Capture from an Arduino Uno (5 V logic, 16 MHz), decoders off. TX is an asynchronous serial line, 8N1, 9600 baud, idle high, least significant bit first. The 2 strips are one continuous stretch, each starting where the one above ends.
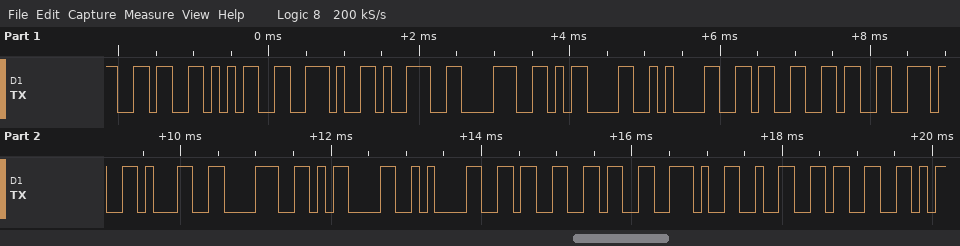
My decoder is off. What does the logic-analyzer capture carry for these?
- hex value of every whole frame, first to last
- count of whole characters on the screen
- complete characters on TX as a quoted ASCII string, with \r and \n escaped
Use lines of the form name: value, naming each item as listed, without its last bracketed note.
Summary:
hex value of every whole frame, first to last: 36 35 2E 39 38 0D 0A 36 36 2E 31 38 0D 0A 36 36 2E 32 33
count of whole characters on the screen: 19
complete characters on TX as a quoted ASCII string, with \r and \n escaped: "65.98\r\n66.18\r\n66.23"
